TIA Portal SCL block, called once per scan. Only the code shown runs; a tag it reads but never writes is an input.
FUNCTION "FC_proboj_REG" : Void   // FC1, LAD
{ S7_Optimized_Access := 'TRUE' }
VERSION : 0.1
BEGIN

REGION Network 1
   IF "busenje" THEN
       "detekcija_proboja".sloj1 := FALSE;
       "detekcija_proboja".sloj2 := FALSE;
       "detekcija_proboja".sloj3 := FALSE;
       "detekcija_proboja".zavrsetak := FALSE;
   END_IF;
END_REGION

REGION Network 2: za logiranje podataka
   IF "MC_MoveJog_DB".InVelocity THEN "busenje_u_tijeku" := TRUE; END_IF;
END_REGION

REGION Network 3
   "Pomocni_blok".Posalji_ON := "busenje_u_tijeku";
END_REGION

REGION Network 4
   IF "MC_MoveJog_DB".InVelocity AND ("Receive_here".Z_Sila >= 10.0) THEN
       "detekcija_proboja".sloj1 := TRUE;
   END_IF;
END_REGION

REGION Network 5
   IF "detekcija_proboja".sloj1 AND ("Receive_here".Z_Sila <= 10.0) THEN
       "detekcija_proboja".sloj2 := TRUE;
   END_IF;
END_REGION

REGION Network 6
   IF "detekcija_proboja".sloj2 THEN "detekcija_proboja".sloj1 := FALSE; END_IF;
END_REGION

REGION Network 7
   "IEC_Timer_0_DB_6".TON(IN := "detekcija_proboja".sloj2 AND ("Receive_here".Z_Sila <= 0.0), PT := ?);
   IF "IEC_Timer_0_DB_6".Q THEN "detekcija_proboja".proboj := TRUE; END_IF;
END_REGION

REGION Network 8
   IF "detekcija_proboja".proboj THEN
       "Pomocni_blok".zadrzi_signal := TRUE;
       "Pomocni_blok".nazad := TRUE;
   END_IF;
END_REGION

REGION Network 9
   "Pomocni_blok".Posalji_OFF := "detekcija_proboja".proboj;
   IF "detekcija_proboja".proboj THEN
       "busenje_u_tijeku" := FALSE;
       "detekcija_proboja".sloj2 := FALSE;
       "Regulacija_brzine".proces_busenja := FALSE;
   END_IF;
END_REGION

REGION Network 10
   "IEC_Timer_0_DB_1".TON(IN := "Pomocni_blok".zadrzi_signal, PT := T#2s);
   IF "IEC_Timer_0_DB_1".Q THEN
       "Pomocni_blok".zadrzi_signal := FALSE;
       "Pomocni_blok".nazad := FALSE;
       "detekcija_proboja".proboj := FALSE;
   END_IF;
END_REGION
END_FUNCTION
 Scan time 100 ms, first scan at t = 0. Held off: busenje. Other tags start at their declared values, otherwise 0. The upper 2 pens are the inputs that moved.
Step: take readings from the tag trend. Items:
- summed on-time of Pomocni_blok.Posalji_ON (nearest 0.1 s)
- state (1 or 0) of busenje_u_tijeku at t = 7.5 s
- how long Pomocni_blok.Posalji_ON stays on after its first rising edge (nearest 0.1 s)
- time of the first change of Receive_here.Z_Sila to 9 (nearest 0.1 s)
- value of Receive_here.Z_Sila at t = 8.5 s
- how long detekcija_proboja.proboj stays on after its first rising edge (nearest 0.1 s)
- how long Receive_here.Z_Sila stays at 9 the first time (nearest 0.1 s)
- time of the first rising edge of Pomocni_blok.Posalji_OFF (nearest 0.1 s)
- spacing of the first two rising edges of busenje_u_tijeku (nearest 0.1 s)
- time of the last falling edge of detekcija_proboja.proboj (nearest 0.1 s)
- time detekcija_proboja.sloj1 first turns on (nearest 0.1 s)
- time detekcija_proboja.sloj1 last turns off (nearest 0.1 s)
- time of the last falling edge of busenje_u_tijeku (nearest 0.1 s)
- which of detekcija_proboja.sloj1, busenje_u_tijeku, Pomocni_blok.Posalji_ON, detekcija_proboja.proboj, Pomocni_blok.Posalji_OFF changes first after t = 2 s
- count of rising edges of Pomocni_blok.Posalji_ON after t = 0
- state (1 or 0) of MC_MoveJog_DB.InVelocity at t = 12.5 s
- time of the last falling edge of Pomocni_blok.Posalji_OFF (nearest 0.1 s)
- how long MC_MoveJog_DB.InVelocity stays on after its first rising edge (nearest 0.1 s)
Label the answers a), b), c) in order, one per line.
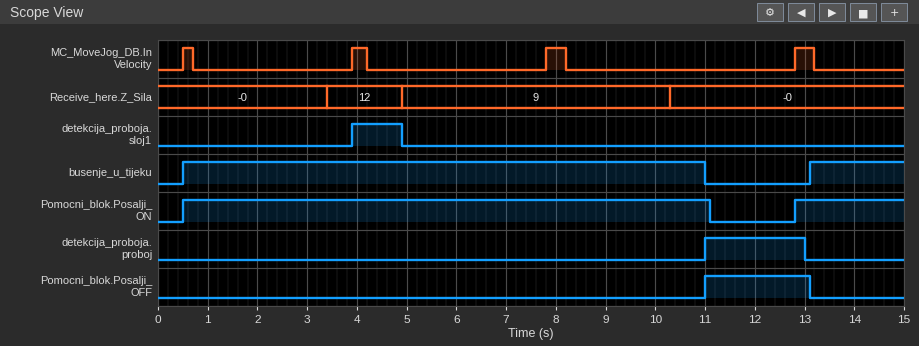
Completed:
a) 12.8 s
b) 1
c) 10.6 s
d) 4.9 s
e) 9
f) 2.0 s
g) 5.4 s
h) 11.0 s
i) 12.6 s
j) 13.0 s
k) 3.9 s
l) 4.9 s
m) 11.0 s
n) detekcija_proboja.sloj1
o) 2
p) 0
q) 13.1 s
r) 0.2 s
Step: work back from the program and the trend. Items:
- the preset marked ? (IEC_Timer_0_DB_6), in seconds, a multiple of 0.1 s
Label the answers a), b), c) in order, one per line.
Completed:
a) 0.7 s
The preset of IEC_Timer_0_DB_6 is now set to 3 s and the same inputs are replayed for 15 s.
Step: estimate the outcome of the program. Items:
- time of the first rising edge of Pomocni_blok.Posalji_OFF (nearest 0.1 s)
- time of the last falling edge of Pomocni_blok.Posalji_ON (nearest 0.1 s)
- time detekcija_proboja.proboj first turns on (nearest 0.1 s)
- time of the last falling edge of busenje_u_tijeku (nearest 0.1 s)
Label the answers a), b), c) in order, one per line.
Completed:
a) 13.3 s
b) 13.4 s
c) 13.3 s
d) 13.3 s
